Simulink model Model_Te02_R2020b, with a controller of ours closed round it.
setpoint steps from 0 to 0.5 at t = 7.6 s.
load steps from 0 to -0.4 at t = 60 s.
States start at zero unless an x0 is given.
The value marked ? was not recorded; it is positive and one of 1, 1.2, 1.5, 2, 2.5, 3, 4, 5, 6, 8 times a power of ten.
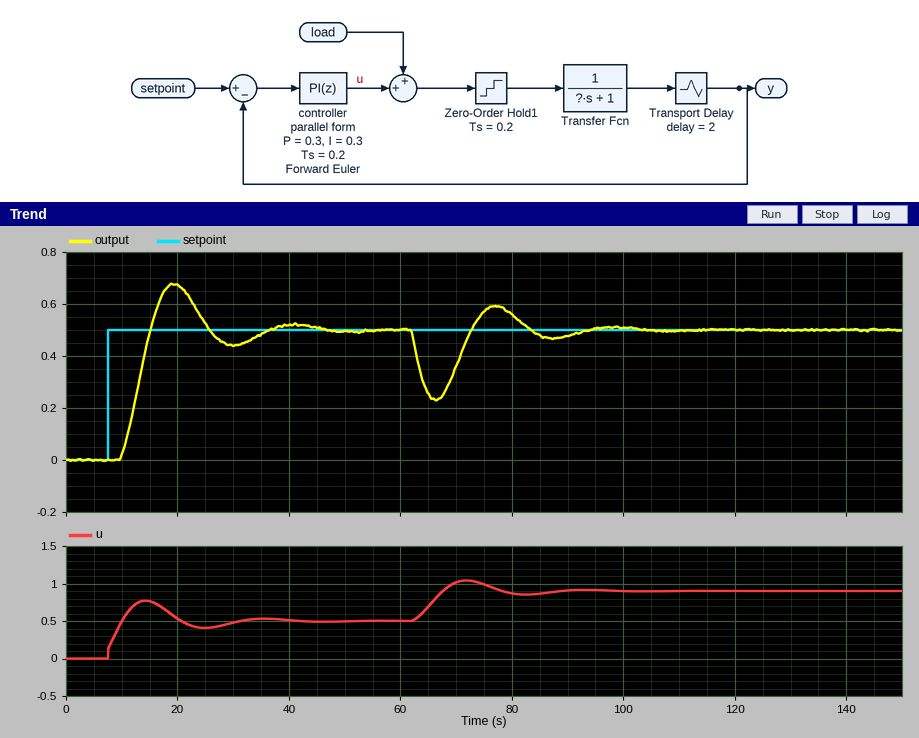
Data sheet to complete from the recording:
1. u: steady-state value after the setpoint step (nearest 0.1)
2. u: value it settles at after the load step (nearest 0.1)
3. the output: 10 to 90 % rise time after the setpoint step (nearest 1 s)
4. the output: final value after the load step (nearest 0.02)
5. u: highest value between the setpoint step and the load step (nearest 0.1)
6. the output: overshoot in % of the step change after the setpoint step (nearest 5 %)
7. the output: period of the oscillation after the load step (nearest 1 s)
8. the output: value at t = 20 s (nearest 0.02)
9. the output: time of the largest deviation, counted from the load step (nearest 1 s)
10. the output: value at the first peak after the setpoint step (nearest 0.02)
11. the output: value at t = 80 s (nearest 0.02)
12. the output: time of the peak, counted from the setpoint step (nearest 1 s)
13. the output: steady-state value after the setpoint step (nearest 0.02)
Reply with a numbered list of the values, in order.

1. 0.5
2. 0.9
3. 4 s
4. 0.50
5. 0.8
6. 35 %
7. 21 s
8. 0.68
9. 6 s
10. 0.68
11. 0.56
12. 12 s
13. 0.50
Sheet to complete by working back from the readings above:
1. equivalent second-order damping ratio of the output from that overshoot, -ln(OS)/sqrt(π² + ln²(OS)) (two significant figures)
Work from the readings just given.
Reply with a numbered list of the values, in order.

1. 0.32
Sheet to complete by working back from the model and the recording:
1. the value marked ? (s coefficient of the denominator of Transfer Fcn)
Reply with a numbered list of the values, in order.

1. 3
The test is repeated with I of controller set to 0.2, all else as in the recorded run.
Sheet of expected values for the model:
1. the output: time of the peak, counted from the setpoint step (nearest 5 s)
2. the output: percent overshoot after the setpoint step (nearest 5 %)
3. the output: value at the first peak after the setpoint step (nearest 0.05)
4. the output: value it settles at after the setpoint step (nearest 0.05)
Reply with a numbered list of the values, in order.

1. 15 s
2. 15 %
3. 0.55
4. 0.50
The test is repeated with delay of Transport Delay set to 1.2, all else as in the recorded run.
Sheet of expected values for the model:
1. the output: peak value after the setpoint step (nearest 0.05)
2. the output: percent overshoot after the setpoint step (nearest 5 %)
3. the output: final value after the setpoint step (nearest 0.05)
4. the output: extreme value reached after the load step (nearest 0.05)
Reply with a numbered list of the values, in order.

1. 0.60
2. 20 %
3. 0.50
4. 0.25
